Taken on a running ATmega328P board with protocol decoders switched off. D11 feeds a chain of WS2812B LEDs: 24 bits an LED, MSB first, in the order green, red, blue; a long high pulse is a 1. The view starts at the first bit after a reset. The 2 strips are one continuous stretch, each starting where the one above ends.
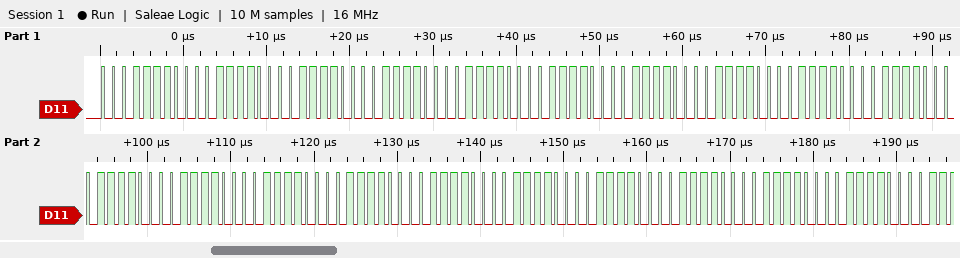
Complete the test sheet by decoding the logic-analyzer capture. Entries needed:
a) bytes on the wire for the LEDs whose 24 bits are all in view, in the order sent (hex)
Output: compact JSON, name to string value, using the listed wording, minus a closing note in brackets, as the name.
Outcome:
{"bytes on the wire for the LEDs whose 24 bits are all in view, in the order sent": "1E 1E 1E 1E 1E 1E 1E 1E 1E 1E 1E 1E 1E 1E 1E 1E 1E 1E"}
